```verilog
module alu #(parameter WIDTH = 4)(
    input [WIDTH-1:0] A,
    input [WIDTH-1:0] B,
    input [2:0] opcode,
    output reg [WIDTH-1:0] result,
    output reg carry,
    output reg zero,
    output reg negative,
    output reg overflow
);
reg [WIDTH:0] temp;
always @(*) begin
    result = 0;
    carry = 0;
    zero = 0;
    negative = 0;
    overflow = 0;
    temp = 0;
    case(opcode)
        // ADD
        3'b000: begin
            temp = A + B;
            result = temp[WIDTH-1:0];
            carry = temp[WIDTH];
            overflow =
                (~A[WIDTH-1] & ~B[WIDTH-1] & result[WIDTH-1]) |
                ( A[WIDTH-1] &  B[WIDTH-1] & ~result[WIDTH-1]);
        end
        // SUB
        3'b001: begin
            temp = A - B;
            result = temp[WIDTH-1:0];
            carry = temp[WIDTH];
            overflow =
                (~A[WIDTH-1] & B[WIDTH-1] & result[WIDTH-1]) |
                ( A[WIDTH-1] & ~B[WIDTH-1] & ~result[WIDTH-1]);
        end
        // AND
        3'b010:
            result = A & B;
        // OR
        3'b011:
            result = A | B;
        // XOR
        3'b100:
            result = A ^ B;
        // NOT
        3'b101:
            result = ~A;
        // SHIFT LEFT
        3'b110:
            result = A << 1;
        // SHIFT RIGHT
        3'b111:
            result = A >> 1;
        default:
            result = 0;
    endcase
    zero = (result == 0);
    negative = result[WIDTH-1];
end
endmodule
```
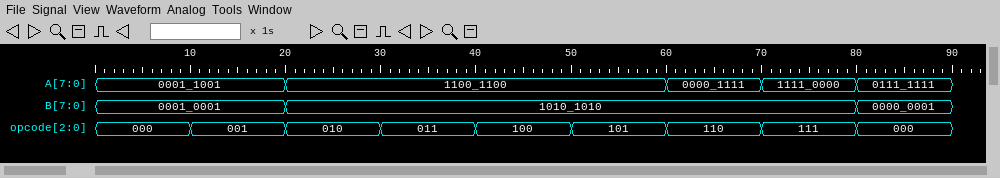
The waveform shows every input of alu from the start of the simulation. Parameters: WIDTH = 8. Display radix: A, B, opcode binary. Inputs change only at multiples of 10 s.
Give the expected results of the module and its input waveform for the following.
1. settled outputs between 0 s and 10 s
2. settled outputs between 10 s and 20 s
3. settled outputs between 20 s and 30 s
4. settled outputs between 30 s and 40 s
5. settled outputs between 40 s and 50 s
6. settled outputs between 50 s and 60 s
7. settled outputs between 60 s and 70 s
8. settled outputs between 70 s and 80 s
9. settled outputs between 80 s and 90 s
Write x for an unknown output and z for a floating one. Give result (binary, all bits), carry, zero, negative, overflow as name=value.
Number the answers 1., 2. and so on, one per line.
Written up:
1. result=00101010, carry=0, zero=0, negative=0, overflow=0
2. result=00001000, carry=0, zero=0, negative=0, overflow=0
3. result=10001000, carry=0, zero=0, negative=1, overflow=0
4. result=11101110, carry=0, zero=0, negative=1, overflow=0
5. result=01100110, carry=0, zero=0, negative=0, overflow=0
6. result=00110011, carry=0, zero=0, negative=0, overflow=0
7. result=00011110, carry=0, zero=0, negative=0, overflow=0
8. result=01111000, carry=0, zero=0, negative=0, overflow=0
9. result=10000000, carry=0, zero=0, negative=1, overflow=1
